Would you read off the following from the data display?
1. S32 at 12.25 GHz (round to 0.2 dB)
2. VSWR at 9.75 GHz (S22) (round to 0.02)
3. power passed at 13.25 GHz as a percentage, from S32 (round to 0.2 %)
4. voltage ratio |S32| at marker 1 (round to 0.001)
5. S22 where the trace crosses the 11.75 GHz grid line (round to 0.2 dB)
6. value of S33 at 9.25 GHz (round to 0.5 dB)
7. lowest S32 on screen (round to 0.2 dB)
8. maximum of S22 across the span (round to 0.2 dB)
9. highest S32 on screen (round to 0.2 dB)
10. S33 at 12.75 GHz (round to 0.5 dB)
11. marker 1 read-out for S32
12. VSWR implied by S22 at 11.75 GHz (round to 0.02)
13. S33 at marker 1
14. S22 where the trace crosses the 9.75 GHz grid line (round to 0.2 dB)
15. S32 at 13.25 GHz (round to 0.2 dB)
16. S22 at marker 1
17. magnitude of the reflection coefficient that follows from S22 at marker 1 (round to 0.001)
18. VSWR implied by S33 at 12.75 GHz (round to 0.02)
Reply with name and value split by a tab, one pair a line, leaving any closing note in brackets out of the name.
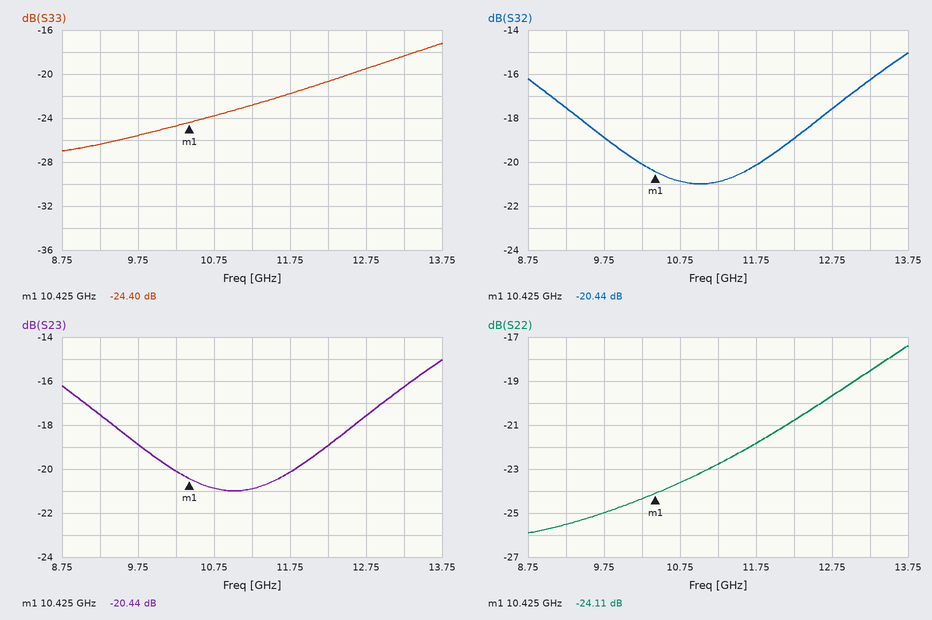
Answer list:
S32 at 12.25 GHz	-19.0 dB
VSWR at 9.75 GHz (S22)	1.12
power passed at 13.25 GHz as a percentage, from S32	2.4 %
voltage ratio |S32| at marker 1	0.095
S22 where the trace crosses the 11.75 GHz grid line	-21.8 dB
value of S33 at 9.25 GHz	-26.5 dB
lowest S32 on screen	-21.0 dB
maximum of S22 across the span	-17.4 dB
highest S32 on screen	-15.0 dB
S33 at 12.75 GHz	-19.5 dB
marker 1 read-out for S32	-20.44 dB
VSWR implied by S22 at 11.75 GHz	1.18
S33 at marker 1	-24.40 dB
S22 where the trace crosses the 9.75 GHz grid line	-25.0 dB
S32 at 13.25 GHz	-16.2 dB
S22 at marker 1	-24.11 dB
magnitude of the reflection coefficient that follows from S22 at marker 1	0.062
VSWR implied by S33 at 12.75 GHz	1.24
